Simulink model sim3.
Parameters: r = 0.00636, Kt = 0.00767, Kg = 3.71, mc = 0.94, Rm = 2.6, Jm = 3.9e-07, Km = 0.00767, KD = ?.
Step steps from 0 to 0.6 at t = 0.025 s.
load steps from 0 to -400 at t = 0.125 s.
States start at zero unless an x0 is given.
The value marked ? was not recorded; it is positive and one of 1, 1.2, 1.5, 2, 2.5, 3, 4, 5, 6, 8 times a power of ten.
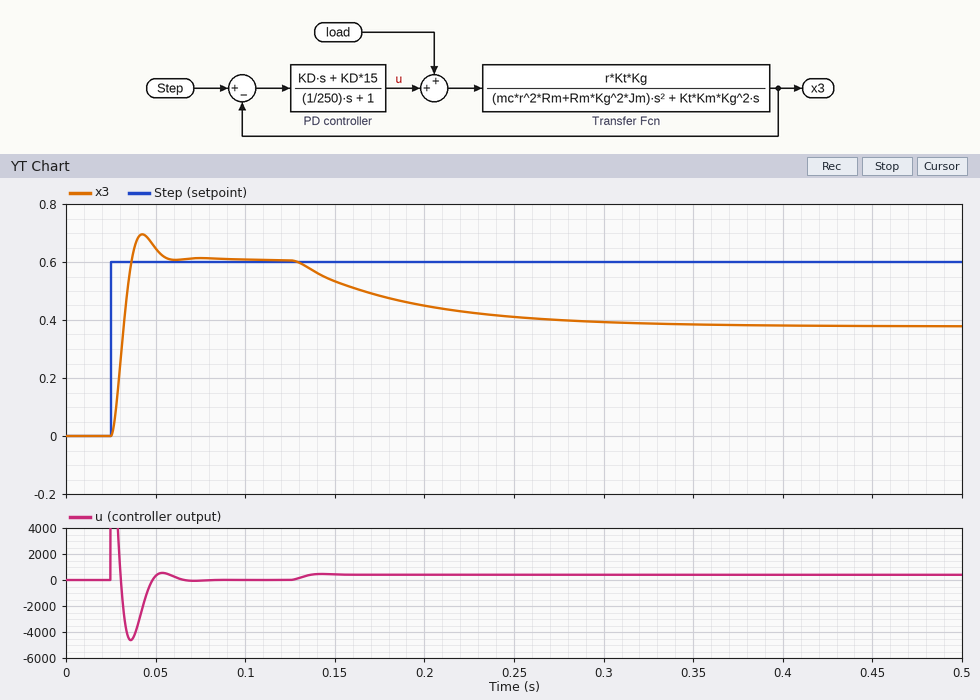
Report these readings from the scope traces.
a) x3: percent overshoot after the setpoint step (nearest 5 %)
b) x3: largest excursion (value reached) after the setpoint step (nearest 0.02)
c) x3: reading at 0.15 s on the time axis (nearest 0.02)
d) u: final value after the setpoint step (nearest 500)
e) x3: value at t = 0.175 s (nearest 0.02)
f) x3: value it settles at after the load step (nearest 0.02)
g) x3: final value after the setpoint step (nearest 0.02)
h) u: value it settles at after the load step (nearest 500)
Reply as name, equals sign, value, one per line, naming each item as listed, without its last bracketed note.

x3: percent overshoot after the setpoint step = 15 %
x3: largest excursion (value reached) after the setpoint step = 0.70
x3: reading at 0.15 s on the time axis = 0.54
u: final value after the setpoint step = 0
x3: value at t = 0.175 s = 0.48
x3: value it settles at after the load step = 0.38
x3: final value after the setpoint step = 0.60
u: value it settles at after the load step = 500
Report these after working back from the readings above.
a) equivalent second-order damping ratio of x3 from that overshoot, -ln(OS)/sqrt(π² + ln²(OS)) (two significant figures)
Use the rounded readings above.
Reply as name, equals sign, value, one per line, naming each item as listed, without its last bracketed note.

equivalent second-order damping ratio of x3 from that overshoot, -ln(OS)/sqrt(π² + ln²(OS)) = 0.52
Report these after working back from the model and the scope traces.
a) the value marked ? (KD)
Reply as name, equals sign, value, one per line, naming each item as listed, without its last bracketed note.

the value marked ? = 120
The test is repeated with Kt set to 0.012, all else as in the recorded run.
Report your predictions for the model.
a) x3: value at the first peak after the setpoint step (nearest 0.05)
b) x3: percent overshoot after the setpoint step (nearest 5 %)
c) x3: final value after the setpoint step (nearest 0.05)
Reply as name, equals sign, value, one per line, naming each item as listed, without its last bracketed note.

x3: value at the first peak after the setpoint step = 0.75
x3: percent overshoot after the setpoint step = 20 %
x3: final value after the setpoint step = 0.60
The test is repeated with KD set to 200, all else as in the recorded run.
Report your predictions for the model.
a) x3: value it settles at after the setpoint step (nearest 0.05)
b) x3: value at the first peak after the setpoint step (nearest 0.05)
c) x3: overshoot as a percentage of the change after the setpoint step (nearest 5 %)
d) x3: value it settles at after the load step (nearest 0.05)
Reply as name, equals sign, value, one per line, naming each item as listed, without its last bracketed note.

x3: value it settles at after the setpoint step = 0.60
x3: value at the first peak after the setpoint step = 0.75
x3: overshoot as a percentage of the change after the setpoint step = 25 %
x3: value it settles at after the load step = 0.45
